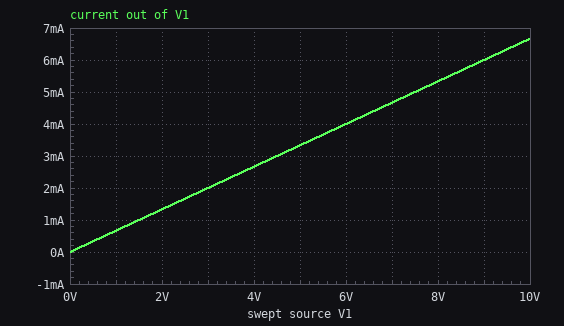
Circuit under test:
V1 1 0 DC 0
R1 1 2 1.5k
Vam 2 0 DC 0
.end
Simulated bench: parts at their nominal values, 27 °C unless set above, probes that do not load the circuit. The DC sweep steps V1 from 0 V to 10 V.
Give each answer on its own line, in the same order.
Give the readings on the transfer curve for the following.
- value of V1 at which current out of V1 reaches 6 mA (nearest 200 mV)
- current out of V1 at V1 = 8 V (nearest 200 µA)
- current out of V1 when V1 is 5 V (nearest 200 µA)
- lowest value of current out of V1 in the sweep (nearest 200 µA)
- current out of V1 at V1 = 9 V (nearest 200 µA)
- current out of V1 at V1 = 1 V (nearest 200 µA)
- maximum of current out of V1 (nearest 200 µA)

9.0 V
5.4 mA
3.4 mA
0 A
6.0 mA
600 µA
6.6 mA
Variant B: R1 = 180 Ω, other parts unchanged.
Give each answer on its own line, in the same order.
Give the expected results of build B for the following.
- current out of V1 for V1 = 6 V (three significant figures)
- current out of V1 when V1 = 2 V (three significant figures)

33.3 mA
11.1 mA
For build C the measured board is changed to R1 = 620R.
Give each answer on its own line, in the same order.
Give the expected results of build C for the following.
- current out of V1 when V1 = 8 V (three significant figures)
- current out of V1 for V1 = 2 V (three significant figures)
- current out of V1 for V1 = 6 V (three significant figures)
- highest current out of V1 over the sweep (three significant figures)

12.9 mA
3.23 mA
9.68 mA
16.1 mA
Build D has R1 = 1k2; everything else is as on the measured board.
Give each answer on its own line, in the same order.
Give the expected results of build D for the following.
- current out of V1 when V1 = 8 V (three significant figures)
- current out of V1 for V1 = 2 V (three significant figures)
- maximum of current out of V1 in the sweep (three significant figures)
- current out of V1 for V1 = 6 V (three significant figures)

6.67 mA
1.67 mA
8.33 mA
5.00 mA
